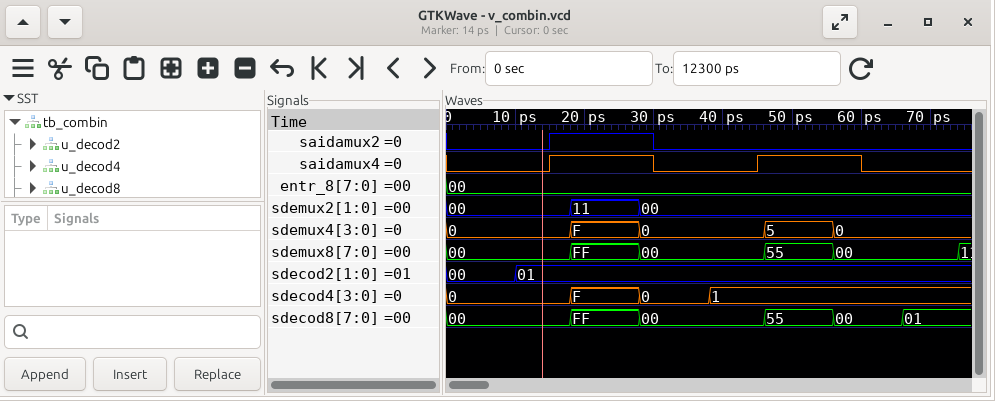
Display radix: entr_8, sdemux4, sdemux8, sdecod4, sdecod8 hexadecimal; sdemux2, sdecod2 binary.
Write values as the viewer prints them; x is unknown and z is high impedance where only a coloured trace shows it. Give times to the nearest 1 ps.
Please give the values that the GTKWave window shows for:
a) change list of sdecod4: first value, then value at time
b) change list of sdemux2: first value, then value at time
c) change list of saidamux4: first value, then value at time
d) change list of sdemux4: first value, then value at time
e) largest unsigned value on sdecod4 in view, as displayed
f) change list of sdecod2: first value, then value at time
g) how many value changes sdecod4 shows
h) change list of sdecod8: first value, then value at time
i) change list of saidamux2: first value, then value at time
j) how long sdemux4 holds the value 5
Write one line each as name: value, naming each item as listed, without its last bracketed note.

change list of sdecod4: first value, then value at time: 0, F at 18 ps, 0 at 28 ps, 1 at 38 ps
change list of sdemux2: first value, then value at time: 00, 11 at 18 ps, 00 at 28 ps
change list of saidamux4: first value, then value at time: 0, 1 at 15 ps, 0 at 30 ps, 1 at 45 ps, 0 at 60 ps
change list of sdemux4: first value, then value at time: 0, F at 18 ps, 0 at 28 ps, 5 at 46 ps, 0 at 56 ps
largest unsigned value on sdecod4 in view, as displayed: F
change list of sdecod2: first value, then value at time: 00, 01 at 10 ps
how many value changes sdecod4 shows: 3
change list of sdecod8: first value, then value at time: 00, FF at 18 ps, 00 at 28 ps, 55 at 46 ps, 00 at 56 ps, 01 at 66 ps
change list of saidamux2: first value, then value at time: 0, 1 at 15 ps, 0 at 30 ps
how long sdemux4 holds the value 5: 10 ps
